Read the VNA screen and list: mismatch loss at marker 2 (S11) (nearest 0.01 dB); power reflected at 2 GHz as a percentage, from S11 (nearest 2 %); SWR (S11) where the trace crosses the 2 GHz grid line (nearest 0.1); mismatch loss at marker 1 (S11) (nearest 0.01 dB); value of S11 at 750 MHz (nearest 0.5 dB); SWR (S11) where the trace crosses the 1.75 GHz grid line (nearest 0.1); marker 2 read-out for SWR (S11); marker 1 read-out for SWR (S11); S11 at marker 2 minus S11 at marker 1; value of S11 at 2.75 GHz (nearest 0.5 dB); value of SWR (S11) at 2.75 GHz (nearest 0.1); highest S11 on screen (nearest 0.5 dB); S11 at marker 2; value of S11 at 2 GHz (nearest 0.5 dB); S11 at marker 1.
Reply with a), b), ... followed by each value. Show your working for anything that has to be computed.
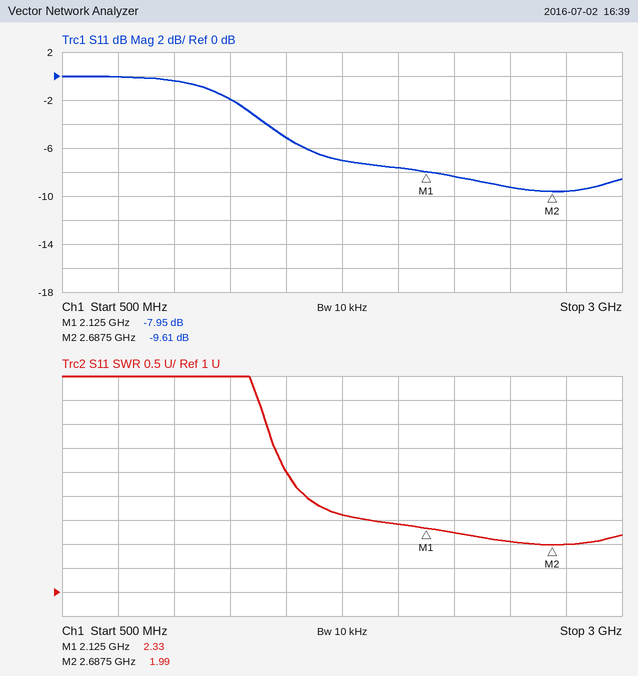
a) −10 log10(1 − 10^(-9.61/10)) ≈ 0.50 dB
b) 10^(-7.5/10) ≈ 18 %
c) 2.4
d) −10 log10(1 − 10^(-7.95/10)) ≈ 0.76 dB
e) 0.0 dB
f) 2.6
g) 1.99
h) 2.33
i) -9.61 − (-7.95) = -1.66 dB
j) -9.5 dB
k) 2.0
l) 0.0 dB
m) -9.61 dB
n) -7.5 dB
o) -7.95 dB
